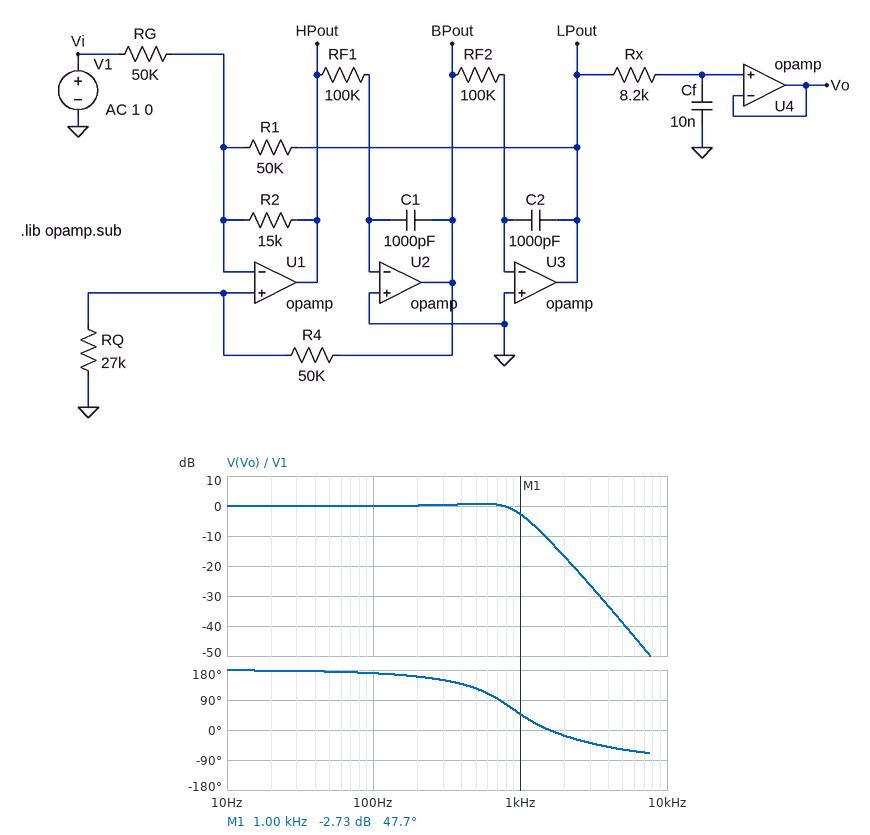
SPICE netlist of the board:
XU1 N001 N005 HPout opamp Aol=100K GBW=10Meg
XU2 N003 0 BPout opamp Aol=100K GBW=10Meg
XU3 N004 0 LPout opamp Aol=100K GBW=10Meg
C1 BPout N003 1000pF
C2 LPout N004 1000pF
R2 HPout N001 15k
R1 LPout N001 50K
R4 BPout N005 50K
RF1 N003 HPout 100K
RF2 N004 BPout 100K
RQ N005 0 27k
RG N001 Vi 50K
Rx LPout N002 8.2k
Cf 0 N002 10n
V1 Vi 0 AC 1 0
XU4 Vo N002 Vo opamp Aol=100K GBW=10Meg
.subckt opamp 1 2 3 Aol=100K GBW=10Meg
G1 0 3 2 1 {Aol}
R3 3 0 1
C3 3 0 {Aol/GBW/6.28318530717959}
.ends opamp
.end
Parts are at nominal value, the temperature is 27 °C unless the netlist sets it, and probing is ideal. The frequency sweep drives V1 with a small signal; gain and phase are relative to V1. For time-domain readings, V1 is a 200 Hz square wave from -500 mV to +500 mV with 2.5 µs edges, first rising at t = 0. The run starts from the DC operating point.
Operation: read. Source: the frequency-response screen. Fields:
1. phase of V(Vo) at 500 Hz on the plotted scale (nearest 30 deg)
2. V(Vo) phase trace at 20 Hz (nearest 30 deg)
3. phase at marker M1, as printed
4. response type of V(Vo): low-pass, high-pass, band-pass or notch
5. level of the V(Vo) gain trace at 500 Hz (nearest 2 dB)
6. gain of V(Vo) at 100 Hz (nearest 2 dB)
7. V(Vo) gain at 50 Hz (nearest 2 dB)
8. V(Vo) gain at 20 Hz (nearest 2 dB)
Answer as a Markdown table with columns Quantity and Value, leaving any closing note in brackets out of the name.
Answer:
| Quantity | Value |
|---|---|
| phase of V(Vo) at 500 Hz on the plotted scale | 120 deg |
| V(Vo) phase trace at 20 Hz | 180 deg |
| phase at marker M1, as printed | 47.7 deg |
| response type of V(Vo): low-pass, high-pass, band-pass or notch | low-pass |
| level of the V(Vo) gain trace at 500 Hz | 0 dB |
| gain of V(Vo) at 100 Hz | 0 dB |
| V(Vo) gain at 50 Hz | 0 dB |
| V(Vo) gain at 20 Hz | 0 dB |
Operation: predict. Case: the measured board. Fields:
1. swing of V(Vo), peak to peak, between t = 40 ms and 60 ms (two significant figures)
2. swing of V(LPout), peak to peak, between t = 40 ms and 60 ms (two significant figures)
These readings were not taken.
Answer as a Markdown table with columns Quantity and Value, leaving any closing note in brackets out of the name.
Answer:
| Quantity | Value |
|---|---|
| swing of V(Vo), peak to peak, between t = 40 ms and 60 ms | 1.3 V |
| swing of V(LPout), peak to peak, between t = 40 ms and 60 ms | 1.3 V |
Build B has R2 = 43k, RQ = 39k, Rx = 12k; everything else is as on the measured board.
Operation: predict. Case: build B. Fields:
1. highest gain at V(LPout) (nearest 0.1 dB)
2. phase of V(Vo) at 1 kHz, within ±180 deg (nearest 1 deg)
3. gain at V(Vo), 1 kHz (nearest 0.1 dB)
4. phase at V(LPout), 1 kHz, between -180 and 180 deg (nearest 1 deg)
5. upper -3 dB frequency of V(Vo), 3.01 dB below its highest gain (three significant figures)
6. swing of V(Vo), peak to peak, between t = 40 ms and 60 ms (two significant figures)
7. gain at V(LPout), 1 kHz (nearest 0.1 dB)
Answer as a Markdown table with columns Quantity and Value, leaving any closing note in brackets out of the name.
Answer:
| Quantity | Value |
|---|---|
| highest gain at V(LPout) | 0.1 dB |
| phase of V(Vo) at 1 kHz, within ±180 deg | 85 deg |
| gain at V(Vo), 1 kHz | -2.2 dB |
| phase at V(LPout), 1 kHz, between -180 and 180 deg | 122 deg |
| upper -3 dB frequency of V(Vo), 3.01 dB below its highest gain | 1.14 kHz |
| swing of V(Vo), peak to peak, between t = 40 ms and 60 ms | 1.0 V |
| gain at V(LPout), 1 kHz | -0.2 dB |
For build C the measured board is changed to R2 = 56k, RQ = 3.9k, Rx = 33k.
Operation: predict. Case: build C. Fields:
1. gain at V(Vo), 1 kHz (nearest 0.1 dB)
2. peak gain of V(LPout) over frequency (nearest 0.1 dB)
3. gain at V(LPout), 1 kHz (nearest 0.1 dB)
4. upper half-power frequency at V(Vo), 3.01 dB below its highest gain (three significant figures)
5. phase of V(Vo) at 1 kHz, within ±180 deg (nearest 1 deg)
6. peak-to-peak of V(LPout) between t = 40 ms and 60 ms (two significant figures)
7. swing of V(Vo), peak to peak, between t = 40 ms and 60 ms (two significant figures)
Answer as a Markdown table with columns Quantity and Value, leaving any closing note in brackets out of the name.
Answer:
| Quantity | Value |
|---|---|
| gain at V(Vo), 1 kHz | -3.6 dB |
| peak gain of V(LPout) over frequency | 13.2 dB |
| gain at V(LPout), 1 kHz | 3.6 dB |
| upper half-power frequency at V(Vo), 3.01 dB below its highest gain | 1.81 kHz |
| phase of V(Vo) at 1 kHz, within ±180 deg | 104 deg |
| peak-to-peak of V(LPout) between t = 40 ms and 60 ms | 2.4 V |
| swing of V(Vo), peak to peak, between t = 40 ms and 60 ms | 1.1 V |
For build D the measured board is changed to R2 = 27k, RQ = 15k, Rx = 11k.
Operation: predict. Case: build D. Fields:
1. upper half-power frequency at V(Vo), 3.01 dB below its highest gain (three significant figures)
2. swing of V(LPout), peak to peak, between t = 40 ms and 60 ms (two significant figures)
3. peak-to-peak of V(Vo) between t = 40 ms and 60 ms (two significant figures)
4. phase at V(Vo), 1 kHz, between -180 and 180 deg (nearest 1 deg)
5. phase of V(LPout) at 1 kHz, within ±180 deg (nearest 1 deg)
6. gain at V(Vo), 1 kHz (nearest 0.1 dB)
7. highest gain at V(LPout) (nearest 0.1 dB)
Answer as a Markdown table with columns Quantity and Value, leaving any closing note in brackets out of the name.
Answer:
| Quantity | Value |
|---|---|
| upper half-power frequency at V(Vo), 3.01 dB below its highest gain | 1.32 kHz |
| swing of V(LPout), peak to peak, between t = 40 ms and 60 ms | 1.7 V |
| peak-to-peak of V(Vo) between t = 40 ms and 60 ms | 1.5 V |
| phase at V(Vo), 1 kHz, between -180 and 180 deg | 81 deg |
| phase of V(LPout) at 1 kHz, within ±180 deg | 116 deg |
| gain at V(Vo), 1 kHz | 2.5 dB |
| highest gain at V(LPout) | 4.2 dB |
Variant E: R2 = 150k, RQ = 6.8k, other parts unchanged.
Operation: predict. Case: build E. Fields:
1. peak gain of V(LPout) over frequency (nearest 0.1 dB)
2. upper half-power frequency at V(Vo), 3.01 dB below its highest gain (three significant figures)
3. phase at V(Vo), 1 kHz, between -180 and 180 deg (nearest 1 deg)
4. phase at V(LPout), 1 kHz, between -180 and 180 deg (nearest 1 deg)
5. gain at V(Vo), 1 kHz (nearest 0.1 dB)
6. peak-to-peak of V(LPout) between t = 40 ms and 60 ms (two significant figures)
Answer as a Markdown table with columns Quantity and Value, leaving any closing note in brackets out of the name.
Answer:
| Quantity | Value |
|---|---|
| peak gain of V(LPout) over frequency | 6.6 dB |
| upper half-power frequency at V(Vo), 3.01 dB below its highest gain | 3.06 kHz |
| phase at V(Vo), 1 kHz, between -180 and 180 deg | 141 deg |
| phase at V(LPout), 1 kHz, between -180 and 180 deg | 169 deg |
| gain at V(Vo), 1 kHz | 0 dB |
| peak-to-peak of V(LPout) between t = 40 ms and 60 ms | 1.9 V |
